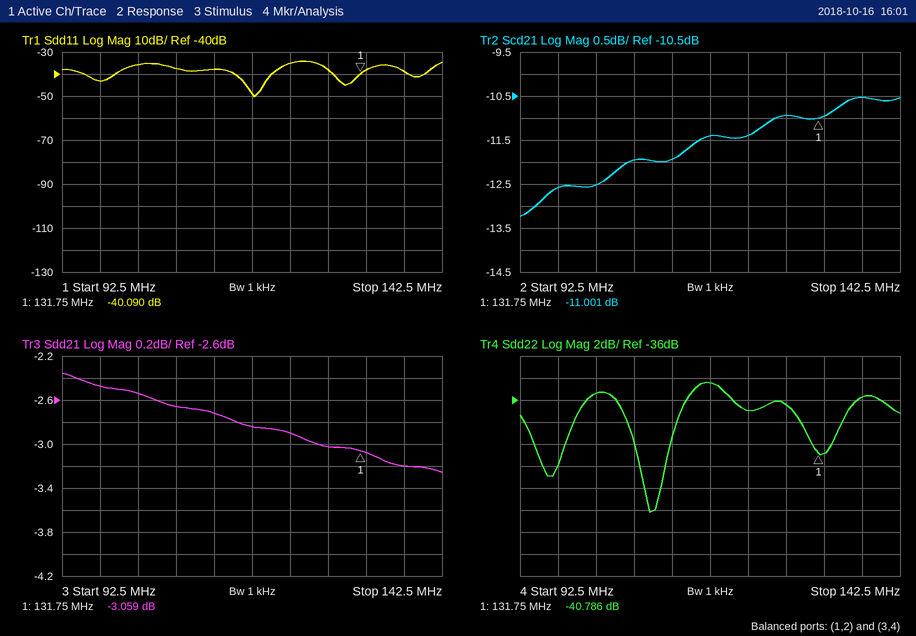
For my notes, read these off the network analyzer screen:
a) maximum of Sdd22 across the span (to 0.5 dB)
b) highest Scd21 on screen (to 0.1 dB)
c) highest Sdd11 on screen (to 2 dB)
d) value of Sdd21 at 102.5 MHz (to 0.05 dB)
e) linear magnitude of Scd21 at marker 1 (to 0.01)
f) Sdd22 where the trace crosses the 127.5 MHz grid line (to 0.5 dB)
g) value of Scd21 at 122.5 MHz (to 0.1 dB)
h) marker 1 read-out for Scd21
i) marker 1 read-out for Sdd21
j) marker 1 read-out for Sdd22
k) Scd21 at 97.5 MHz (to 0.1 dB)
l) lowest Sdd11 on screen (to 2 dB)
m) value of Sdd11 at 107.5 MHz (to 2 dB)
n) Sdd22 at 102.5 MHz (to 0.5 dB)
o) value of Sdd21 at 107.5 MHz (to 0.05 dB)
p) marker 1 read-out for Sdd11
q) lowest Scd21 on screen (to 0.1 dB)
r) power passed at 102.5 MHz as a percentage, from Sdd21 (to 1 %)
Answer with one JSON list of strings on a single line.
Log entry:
["-34.5 dB", "-10.5 dB", "-34 dB", "-2.55 dB", "0.28", "-36.5 dB", "-11.4 dB", "-11.001 dB", "-3.059 dB", "-40.786 dB", "-12.6 dB", "-50 dB", "-38 dB", "-35.5 dB", "-2.65 dB", "-40.090 dB", "-13.2 dB", "56 %"]
